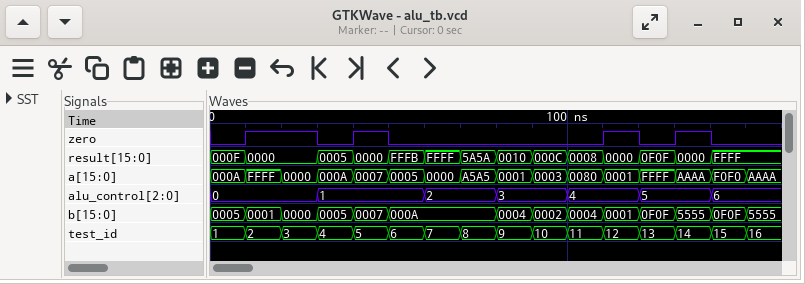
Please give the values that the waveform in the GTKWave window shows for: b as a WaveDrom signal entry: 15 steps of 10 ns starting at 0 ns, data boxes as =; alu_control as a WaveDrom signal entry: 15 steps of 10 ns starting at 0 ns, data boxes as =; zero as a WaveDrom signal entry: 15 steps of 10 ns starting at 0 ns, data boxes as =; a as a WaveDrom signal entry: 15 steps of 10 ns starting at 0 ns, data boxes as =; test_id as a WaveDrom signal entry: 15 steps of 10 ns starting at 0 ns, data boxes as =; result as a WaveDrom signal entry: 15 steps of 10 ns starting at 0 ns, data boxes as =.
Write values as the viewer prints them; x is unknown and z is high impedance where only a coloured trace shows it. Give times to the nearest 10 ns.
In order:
{name: 'b', wave: '======..=======', data: '0005 0001 0000 0005 0007 000A 0004 0002 0004 0001 0F0F 5555 0F0F'}
{name: 'alu_control', wave: '=..=..=.=.=.=.=', data: '0 1 2 3 4 5 6'}
{name: 'zero', wave: '01.010.....1010'}
{name: 'a', wave: '===============', data: '000A FFFF 0000 000A 0007 0005 0000 A5A5 0001 0003 0080 0001 FFFF AAAA F0F0'}
{name: 'test_id', wave: '===============', data: '1 2 3 4 5 6 7 8 9 10 11 12 13 14 15'}
{name: 'result', wave: '==.============', data: '000F 0000 0005 0000 FFFB FFFF 5A5A 0010 000C 0008 0000 0F0F 0000 FFFF'}
